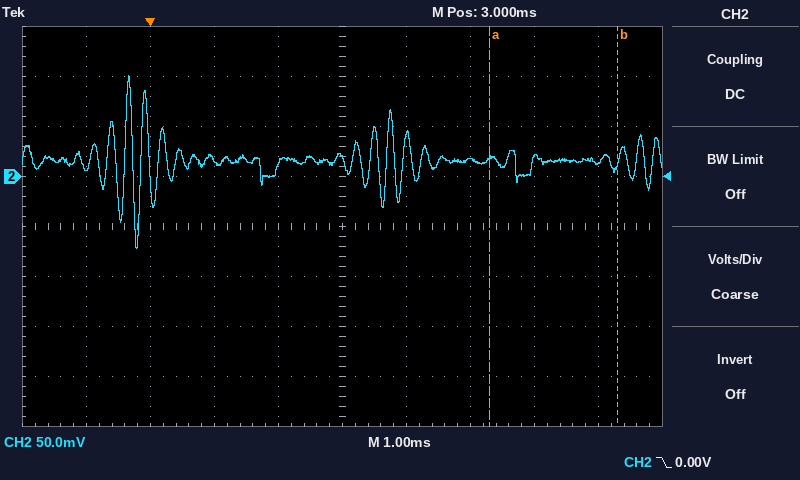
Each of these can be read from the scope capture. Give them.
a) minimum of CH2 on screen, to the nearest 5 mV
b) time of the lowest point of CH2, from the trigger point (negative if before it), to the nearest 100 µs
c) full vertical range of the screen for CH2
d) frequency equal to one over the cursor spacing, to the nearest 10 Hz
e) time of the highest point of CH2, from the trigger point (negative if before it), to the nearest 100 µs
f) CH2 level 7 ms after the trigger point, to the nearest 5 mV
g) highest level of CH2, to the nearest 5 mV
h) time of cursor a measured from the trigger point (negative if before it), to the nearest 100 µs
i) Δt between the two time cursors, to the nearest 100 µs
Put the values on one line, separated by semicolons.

-70 mV; -200 µs; 400 mV; 500 Hz; -300 µs; 15 mV; 100 mV; +5.3 ms; 2.0 ms
